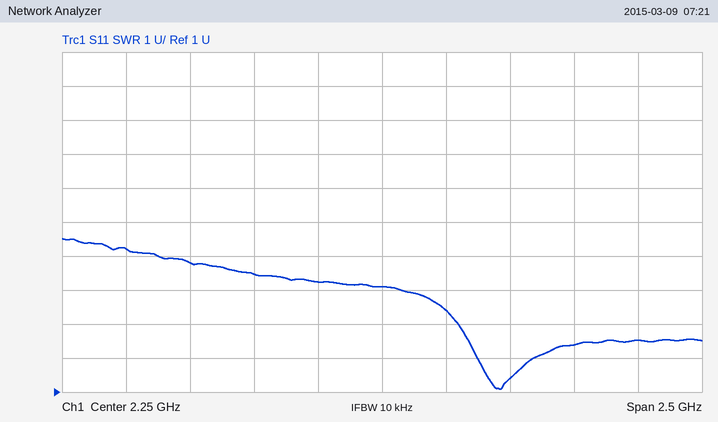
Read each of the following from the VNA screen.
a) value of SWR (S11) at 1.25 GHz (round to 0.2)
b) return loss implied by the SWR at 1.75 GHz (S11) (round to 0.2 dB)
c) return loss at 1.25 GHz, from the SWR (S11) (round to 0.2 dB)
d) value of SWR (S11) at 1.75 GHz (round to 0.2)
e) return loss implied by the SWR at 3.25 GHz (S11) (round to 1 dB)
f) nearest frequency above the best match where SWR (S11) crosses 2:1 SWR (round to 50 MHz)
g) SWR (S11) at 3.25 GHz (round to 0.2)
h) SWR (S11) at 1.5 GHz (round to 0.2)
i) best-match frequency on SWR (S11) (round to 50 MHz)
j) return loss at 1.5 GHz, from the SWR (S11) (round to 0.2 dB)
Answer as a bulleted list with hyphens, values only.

- 5.2
- 4.0 dB
- 3.4 dB
- 4.4
- 7 dB
- 2.85 GHz
- 2.6
- 4.8
- 2.70 GHz
- 3.6 dB
